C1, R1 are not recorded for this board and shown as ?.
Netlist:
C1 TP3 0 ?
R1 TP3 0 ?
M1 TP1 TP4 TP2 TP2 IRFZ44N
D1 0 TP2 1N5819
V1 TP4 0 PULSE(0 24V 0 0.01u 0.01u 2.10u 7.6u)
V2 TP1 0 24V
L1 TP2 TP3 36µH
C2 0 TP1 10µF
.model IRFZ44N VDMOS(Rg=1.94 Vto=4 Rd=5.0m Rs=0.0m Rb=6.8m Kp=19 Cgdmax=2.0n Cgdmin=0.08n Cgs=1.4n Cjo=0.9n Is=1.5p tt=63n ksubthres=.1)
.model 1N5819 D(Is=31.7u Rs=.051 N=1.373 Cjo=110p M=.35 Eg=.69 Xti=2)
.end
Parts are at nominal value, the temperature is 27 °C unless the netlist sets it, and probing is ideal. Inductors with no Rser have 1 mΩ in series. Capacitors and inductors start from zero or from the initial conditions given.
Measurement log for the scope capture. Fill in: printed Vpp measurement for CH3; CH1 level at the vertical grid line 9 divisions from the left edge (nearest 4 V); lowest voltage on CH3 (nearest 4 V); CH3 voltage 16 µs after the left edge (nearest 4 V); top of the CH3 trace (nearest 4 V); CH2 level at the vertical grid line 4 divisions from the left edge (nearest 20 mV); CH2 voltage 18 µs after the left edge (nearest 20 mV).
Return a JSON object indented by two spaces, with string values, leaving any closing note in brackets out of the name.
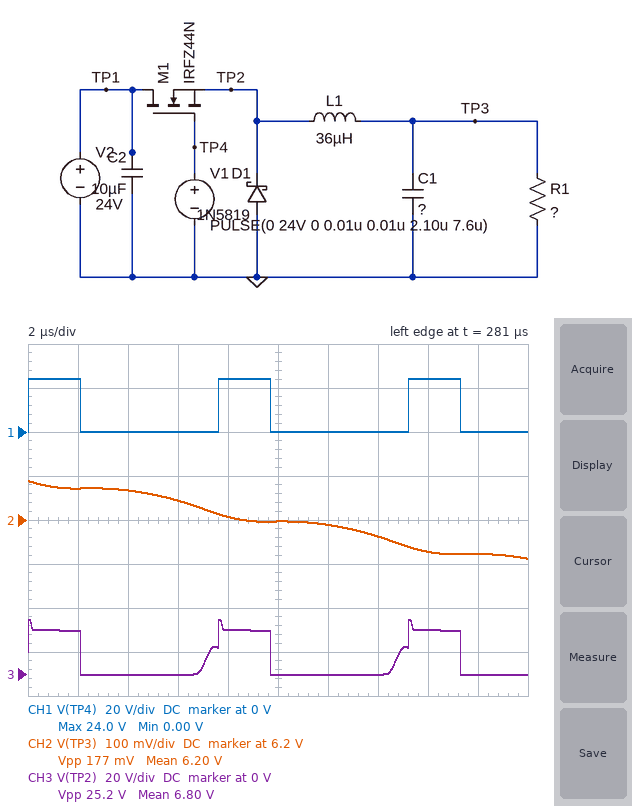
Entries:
{
  "printed Vpp measurement for CH3": "25.2 V",
  "CH1 level at the vertical grid line 9 divisions from the left edge": "0 V",
  "lowest voltage on CH3": "0 V",
  "CH3 voltage 16 µs after the left edge": "20 V",
  "top of the CH3 trace": "24 V",
  "CH2 level at the vertical grid line 4 divisions from the left edge": "6.20 V",
  "CH2 voltage 18 µs after the left edge": "6.12 V"
}
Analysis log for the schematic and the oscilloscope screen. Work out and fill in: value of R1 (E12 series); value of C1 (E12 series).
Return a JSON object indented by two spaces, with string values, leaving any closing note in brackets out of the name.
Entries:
{
  "value of R1": "8.2 Ω",
  "value of C1": "39 µF"
}
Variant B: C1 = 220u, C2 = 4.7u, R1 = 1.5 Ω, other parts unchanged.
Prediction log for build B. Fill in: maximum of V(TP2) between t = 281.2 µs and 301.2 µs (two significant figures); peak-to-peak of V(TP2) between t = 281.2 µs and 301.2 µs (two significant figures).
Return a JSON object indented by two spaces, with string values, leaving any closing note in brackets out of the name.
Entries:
{
  "maximum of V(TP2) between t = 281.2 µs and 301.2 µs": "19 V",
  "peak-to-peak of V(TP2) between t = 281.2 µs and 301.2 µs": "20 V"
}
